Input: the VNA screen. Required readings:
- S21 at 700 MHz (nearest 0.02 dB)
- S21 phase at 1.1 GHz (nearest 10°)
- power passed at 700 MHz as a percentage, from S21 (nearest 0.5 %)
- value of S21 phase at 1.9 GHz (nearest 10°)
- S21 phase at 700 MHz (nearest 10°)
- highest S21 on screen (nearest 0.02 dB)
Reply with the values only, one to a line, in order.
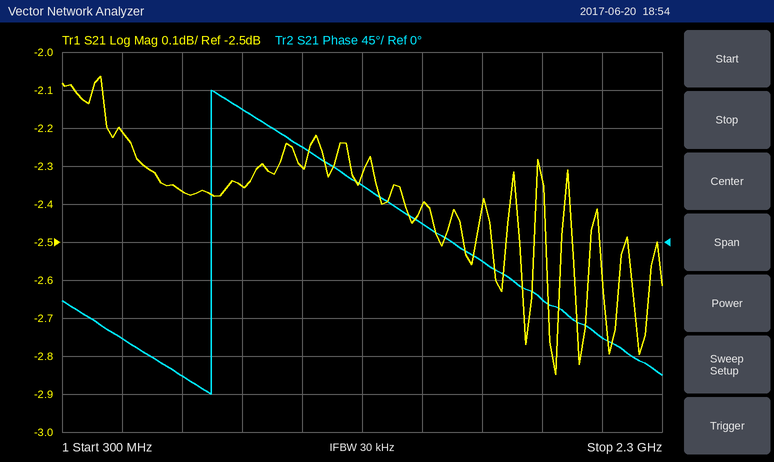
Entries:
-2.36 dB
110°
58.0 %
-70°
-160°
-2.06 dB
